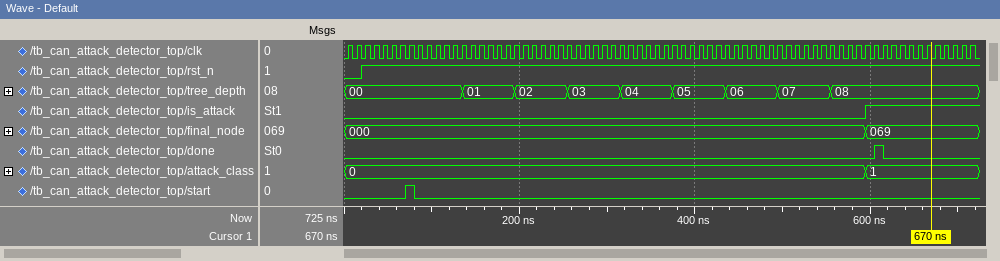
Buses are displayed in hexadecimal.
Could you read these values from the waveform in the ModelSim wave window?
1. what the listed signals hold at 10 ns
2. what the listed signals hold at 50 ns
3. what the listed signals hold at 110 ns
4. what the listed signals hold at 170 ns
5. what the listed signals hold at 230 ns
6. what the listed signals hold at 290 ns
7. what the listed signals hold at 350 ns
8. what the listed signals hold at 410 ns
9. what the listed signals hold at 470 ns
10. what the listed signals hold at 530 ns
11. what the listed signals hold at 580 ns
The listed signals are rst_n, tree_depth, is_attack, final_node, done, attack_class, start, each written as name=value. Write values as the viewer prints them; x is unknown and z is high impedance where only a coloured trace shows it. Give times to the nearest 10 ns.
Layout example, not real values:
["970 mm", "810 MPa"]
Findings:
["rst_n=0, tree_depth=00, is_attack=0, final_node=000, done=0, attack_class=0, start=0", "rst_n=1, tree_depth=00, is_attack=0, final_node=000, done=0, attack_class=0, start=0", "rst_n=1, tree_depth=00, is_attack=0, final_node=000, done=0, attack_class=0, start=0", "rst_n=1, tree_depth=01, is_attack=0, final_node=000, done=0, attack_class=0, start=0", "rst_n=1, tree_depth=02, is_attack=0, final_node=000, done=0, attack_class=0, start=0", "rst_n=1, tree_depth=03, is_attack=0, final_node=000, done=0, attack_class=0, start=0", "rst_n=1, tree_depth=04, is_attack=0, final_node=000, done=0, attack_class=0, start=0", "rst_n=1, tree_depth=05, is_attack=0, final_node=000, done=0, attack_class=0, start=0", "rst_n=1, tree_depth=06, is_attack=0, final_node=000, done=0, attack_class=0, start=0", "rst_n=1, tree_depth=07, is_attack=0, final_node=000, done=0, attack_class=0, start=0", "rst_n=1, tree_depth=08, is_attack=0, final_node=000, done=0, attack_class=0, start=0"]
